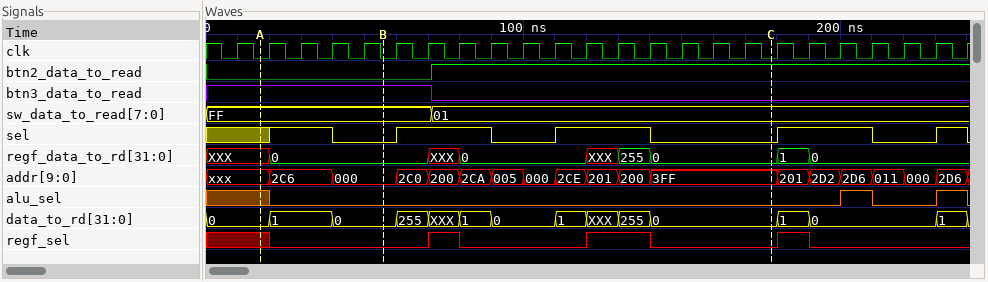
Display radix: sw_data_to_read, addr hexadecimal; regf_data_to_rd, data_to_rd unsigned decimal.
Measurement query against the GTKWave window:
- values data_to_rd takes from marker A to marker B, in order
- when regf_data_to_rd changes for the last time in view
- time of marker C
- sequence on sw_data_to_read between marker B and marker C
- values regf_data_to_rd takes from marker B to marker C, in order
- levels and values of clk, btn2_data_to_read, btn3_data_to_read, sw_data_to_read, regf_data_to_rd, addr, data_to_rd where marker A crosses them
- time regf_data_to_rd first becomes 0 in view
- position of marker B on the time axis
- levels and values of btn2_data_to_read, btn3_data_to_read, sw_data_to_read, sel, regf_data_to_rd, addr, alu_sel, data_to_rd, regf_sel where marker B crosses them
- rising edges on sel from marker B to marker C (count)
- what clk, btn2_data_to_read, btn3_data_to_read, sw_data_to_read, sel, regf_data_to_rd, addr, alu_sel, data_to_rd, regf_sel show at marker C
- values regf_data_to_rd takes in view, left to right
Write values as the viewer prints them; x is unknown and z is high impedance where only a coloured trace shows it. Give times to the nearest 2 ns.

0, 1, 0
190 ns
178 ns
FF, 01
0, XXX, 0, XXX, 255, 0
clk=0, btn2_data_to_read=0, btn3_data_to_read=1, sw_data_to_read=FF, regf_data_to_rd=XXX, addr=xxx, data_to_rd=0
20 ns
56 ns
btn2_data_to_read=0, btn3_data_to_read=1, sw_data_to_read=FF, sel=0, regf_data_to_rd=0, addr=000, alu_sel=0, data_to_rd=0, regf_sel=0
2
clk=0, btn2_data_to_read=1, btn3_data_to_read=0, sw_data_to_read=01, sel=0, regf_data_to_rd=0, addr=3FF, alu_sel=0, data_to_rd=0, regf_sel=0
XXX, 0, XXX, 0, XXX, 255, 0, 1, 0
